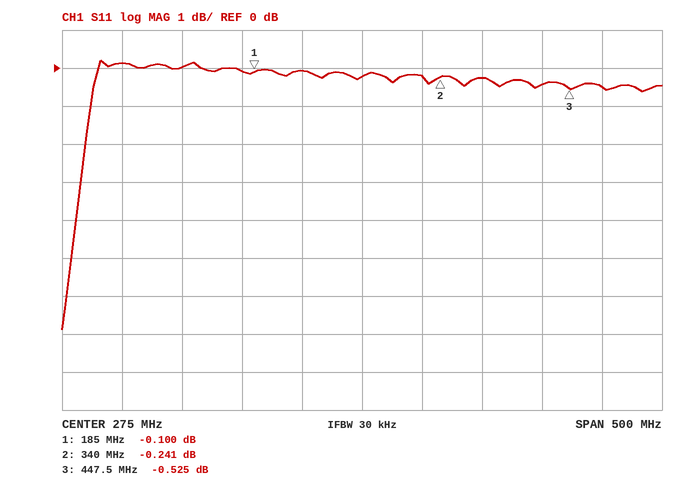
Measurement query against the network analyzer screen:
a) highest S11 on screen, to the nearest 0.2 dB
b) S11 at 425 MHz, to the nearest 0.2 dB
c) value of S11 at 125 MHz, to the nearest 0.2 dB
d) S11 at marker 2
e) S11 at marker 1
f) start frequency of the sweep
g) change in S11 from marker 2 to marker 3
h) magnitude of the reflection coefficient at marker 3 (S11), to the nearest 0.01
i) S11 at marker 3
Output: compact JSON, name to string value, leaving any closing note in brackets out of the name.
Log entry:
{"highest S11 on screen, to the nearest 0.2 dB": "0.2 dB", "S11 at 425 MHz, to the nearest 0.2 dB": "-0.4 dB", "value of S11 at 125 MHz, to the nearest 0.2 dB": "0.0 dB", "S11 at marker 2": "-0.241 dB", "S11 at marker 1": "-0.100 dB", "start frequency of the sweep": "25 MHz", "change in S11 from marker 2 to marker 3": "-0.284 dB", "magnitude of the reflection coefficient at marker 3 (S11), to the nearest 0.01": "0.94", "S11 at marker 3": "-0.525 dB"}
